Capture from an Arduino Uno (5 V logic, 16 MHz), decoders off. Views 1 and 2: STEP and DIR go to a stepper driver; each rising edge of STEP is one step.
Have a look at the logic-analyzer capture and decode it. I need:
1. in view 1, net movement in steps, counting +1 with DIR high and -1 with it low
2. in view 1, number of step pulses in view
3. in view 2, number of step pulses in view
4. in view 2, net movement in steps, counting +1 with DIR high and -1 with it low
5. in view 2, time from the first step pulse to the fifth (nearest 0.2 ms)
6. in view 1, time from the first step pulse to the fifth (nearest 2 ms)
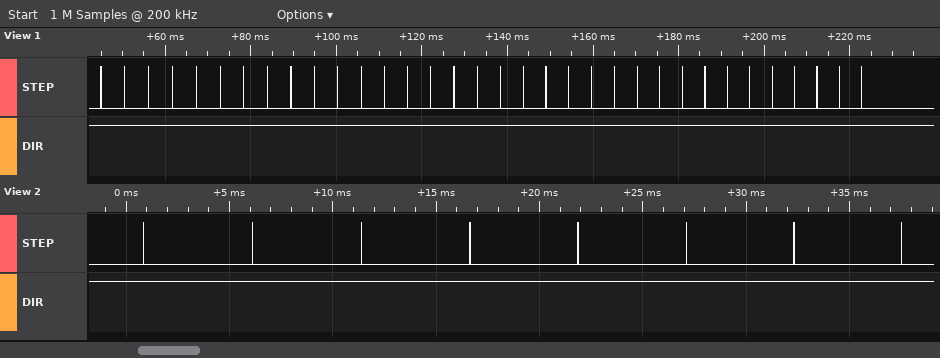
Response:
+34
34
8
+8
21.0 ms
22 ms
